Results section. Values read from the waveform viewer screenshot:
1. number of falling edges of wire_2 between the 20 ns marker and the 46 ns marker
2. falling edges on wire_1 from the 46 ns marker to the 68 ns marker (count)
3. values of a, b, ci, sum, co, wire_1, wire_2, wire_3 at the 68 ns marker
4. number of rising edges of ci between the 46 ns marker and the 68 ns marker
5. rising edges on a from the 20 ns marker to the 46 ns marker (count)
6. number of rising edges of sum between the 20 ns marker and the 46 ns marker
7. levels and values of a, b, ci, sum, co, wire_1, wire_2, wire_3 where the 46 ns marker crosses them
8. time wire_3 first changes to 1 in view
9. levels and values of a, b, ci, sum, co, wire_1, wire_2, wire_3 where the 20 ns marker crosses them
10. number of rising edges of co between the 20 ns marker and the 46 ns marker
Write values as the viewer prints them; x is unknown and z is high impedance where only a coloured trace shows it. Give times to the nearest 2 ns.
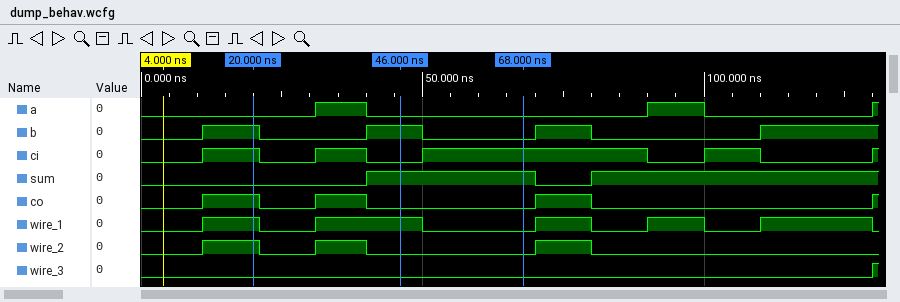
2
1
a=0, b=0, ci=1, sum=1, co=0, wire_1=0, wire_2=0, wire_3=0
1
1
1
a=0, b=1, ci=0, sum=1, co=0, wire_1=1, wire_2=0, wire_3=0
130 ns
a=0, b=1, ci=1, sum=0, co=1, wire_1=1, wire_2=1, wire_3=0
1
